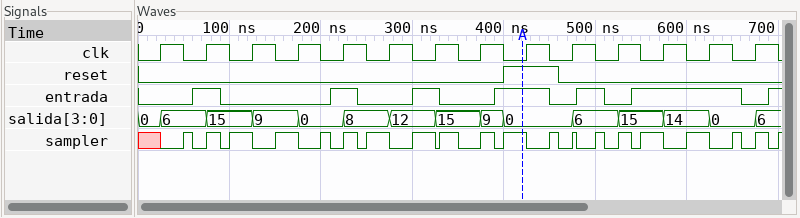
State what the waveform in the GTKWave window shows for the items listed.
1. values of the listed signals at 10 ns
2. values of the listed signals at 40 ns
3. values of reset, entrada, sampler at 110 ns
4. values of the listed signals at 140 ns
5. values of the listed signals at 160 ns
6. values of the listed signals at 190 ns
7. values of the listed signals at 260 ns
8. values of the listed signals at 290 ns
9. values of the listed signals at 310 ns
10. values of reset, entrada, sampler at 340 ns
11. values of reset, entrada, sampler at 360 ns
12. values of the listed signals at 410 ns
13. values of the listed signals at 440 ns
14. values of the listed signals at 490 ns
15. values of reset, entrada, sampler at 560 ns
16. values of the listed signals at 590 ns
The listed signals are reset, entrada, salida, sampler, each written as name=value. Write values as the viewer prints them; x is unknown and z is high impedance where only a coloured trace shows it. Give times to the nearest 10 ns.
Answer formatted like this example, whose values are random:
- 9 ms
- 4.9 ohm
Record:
- reset=0, entrada=0, salida=0, sampler=x
- reset=0, entrada=0, salida=6, sampler=0
- reset=0, entrada=0, sampler=1
- reset=0, entrada=0, salida=9, sampler=0
- reset=0, entrada=0, salida=9, sampler=1
- reset=0, entrada=0, salida=0, sampler=0
- reset=0, entrada=0, salida=8, sampler=1
- reset=0, entrada=0, salida=12, sampler=0
- reset=0, entrada=1, salida=12, sampler=1
- reset=0, entrada=0, sampler=1
- reset=0, entrada=0, sampler=0
- reset=1, entrada=1, salida=0, sampler=1
- reset=1, entrada=1, salida=0, sampler=0
- reset=0, entrada=1, salida=6, sampler=0
- reset=0, entrada=1, sampler=1
- reset=0, entrada=1, salida=14, sampler=0
